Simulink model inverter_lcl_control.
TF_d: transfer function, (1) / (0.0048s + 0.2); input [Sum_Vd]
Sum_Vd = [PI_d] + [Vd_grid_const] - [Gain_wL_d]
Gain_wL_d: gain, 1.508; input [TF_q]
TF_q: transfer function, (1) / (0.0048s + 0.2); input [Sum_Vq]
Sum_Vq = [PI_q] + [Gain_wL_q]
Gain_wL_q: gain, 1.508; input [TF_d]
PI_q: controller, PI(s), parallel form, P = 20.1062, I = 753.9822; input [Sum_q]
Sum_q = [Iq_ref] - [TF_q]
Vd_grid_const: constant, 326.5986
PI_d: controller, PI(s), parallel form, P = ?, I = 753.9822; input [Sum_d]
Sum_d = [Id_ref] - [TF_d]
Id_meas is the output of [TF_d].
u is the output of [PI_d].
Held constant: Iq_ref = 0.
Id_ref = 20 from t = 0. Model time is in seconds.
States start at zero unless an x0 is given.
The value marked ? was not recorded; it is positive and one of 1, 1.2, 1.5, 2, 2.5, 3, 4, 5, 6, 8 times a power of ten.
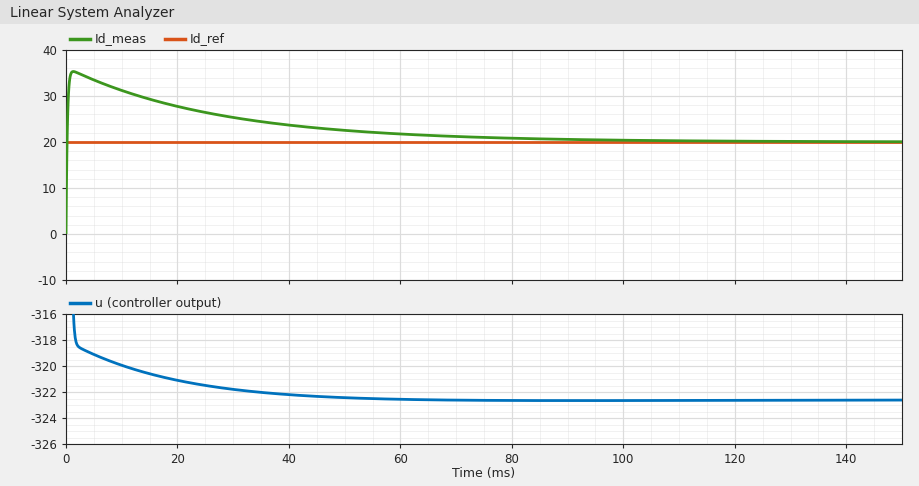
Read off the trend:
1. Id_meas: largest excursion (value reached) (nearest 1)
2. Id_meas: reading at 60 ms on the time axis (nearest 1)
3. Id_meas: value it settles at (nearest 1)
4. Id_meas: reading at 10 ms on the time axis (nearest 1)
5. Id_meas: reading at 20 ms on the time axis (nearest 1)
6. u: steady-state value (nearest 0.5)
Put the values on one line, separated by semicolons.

35; 22; 20; 31; 28; -322.5
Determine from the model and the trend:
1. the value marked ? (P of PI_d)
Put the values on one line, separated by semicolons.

20
